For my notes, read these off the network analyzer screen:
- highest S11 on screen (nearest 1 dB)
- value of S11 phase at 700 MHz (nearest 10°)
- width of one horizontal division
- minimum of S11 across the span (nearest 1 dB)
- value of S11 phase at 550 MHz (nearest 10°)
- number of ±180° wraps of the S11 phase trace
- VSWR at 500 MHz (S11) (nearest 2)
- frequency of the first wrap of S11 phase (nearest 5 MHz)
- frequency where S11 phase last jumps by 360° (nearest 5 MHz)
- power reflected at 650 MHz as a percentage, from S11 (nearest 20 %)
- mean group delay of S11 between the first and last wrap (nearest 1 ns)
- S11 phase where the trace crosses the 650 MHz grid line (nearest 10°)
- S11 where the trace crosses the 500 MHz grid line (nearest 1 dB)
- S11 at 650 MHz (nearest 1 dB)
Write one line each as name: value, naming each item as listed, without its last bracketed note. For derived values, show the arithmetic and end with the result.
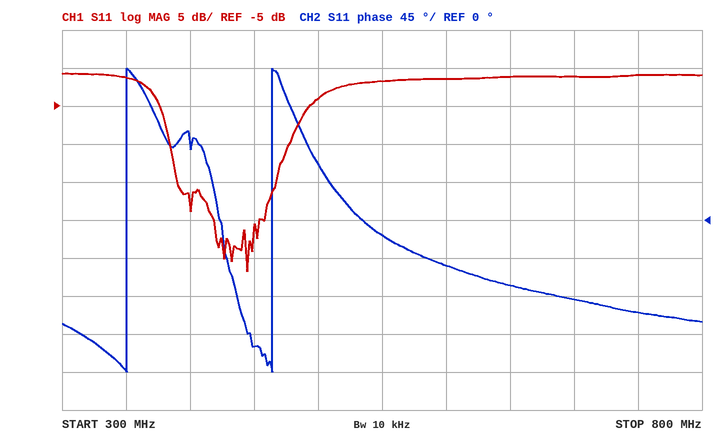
highest S11 on screen: -1 dB
value of S11 phase at 700 MHz: -90°
width of one horizontal division: 50 MHz
minimum of S11 across the span: -27 dB
value of S11 phase at 550 MHz: -20°
number of ±180° wraps of the S11 phase trace: 2
VSWR at 500 MHz (S11): |Γ| = 10^(-4/20) = 0.6310; VSWR = (1 + 0.6310)/(1 − 0.6310) ≈ 4
frequency of the first wrap of S11 phase: 350 MHz
frequency where S11 phase last jumps by 360°: 465 MHz
power reflected at 650 MHz as a percentage, from S11: 10^(-1/10) ≈ 79.4 %, so 80 % to the nearest 20 %
mean group delay of S11 between the first and last wrap: 1 cycle / (465 MHz − 350 MHz) ≈ 9 ns
S11 phase where the trace crosses the 650 MHz grid line: -80°
S11 where the trace crosses the 500 MHz grid line: -4 dB
S11 at 650 MHz: -1 dB
